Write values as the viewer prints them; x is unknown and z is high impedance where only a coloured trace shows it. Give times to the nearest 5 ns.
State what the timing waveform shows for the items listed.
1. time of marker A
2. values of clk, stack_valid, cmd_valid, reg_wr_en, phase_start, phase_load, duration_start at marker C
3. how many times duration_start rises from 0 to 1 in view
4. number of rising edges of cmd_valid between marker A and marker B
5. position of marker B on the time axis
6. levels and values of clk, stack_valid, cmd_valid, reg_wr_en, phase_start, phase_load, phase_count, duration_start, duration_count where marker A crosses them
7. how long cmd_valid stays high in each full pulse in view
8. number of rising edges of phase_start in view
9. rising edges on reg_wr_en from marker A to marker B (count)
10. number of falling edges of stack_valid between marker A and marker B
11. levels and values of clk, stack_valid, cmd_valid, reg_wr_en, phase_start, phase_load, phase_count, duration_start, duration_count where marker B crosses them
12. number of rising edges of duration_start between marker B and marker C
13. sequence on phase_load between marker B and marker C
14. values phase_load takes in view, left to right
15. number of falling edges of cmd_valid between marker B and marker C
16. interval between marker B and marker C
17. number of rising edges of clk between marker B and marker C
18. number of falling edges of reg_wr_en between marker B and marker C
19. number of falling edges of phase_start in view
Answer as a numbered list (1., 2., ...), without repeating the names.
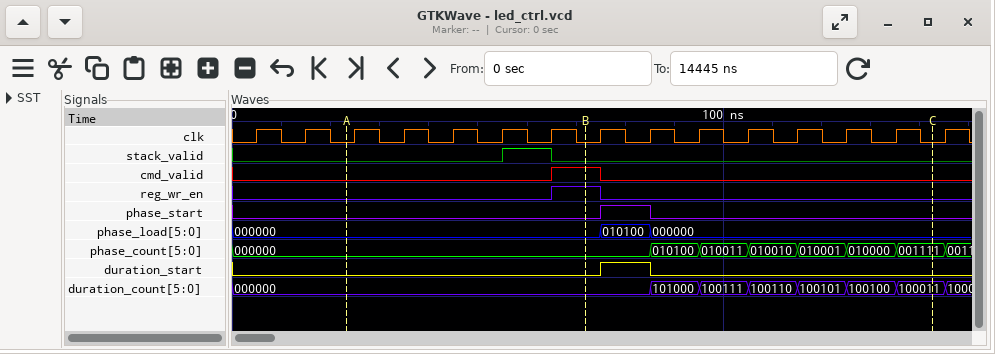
1. 25 ns
2. clk=0, stack_valid=0, cmd_valid=0, reg_wr_en=0, phase_start=0, phase_load=000000, duration_start=0
3. 1
4. 1
5. 70 ns
6. clk=0, stack_valid=0, cmd_valid=0, reg_wr_en=0, phase_start=0, phase_load=000000, phase_count=000000, duration_start=0, duration_count=000000
7. 10 ns
8. 1
9. 1
10. 1
11. clk=0, stack_valid=0, cmd_valid=1, reg_wr_en=1, phase_start=0, phase_load=000000, phase_count=000000, duration_start=0, duration_count=000000
12. 1
13. 000000, 010100, 000000
14. 000000, 010100, 000000
15. 1
16. 70 ns
17. 7
18. 1
19. 1
